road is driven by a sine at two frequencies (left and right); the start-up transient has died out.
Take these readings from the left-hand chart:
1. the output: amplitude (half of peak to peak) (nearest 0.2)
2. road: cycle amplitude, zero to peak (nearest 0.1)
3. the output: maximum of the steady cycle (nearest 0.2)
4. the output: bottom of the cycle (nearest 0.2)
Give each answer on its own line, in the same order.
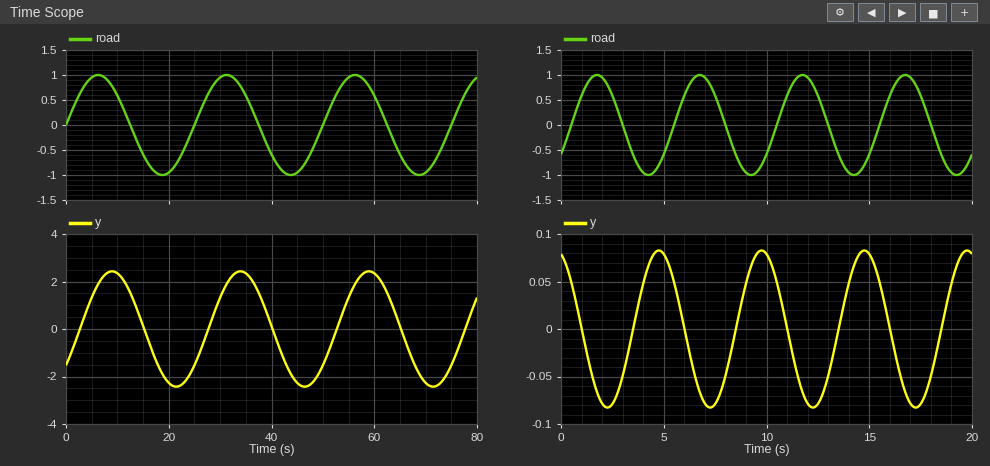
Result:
2.4
1.0
2.4
-2.4
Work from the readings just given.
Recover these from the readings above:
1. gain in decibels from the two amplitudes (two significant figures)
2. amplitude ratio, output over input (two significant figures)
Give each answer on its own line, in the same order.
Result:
7.6 dB
2.4
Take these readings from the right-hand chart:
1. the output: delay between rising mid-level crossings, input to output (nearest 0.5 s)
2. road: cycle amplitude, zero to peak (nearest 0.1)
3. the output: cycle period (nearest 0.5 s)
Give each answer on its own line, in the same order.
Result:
3.0 s
1.0
5.0 s
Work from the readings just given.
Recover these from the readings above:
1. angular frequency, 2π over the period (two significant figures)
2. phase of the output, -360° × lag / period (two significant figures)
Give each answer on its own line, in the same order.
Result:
1.3 rad/s
-220°
